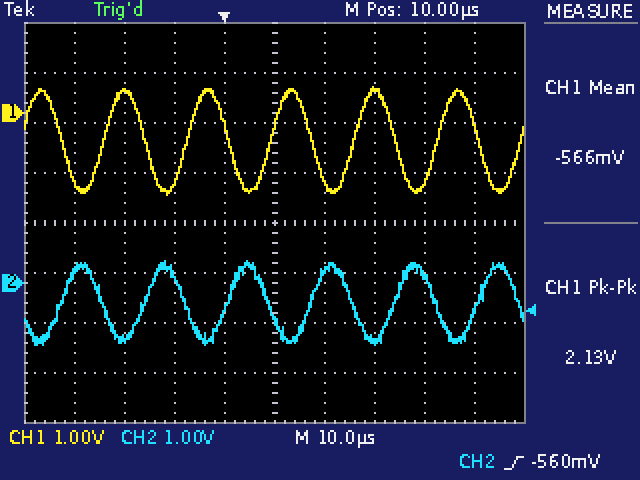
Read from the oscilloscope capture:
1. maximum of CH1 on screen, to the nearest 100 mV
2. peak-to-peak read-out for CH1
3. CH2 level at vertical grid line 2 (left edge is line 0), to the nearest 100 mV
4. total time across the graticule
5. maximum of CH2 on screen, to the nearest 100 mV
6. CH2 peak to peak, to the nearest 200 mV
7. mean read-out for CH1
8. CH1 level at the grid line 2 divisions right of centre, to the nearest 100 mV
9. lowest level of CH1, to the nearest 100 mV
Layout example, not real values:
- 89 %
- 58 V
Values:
- 500 mV
- 2.13 V
- -1.1 V
- 100 µs
- 400 mV
- 1.6 V
- -566 mV
- 400 mV
- -1.6 V
